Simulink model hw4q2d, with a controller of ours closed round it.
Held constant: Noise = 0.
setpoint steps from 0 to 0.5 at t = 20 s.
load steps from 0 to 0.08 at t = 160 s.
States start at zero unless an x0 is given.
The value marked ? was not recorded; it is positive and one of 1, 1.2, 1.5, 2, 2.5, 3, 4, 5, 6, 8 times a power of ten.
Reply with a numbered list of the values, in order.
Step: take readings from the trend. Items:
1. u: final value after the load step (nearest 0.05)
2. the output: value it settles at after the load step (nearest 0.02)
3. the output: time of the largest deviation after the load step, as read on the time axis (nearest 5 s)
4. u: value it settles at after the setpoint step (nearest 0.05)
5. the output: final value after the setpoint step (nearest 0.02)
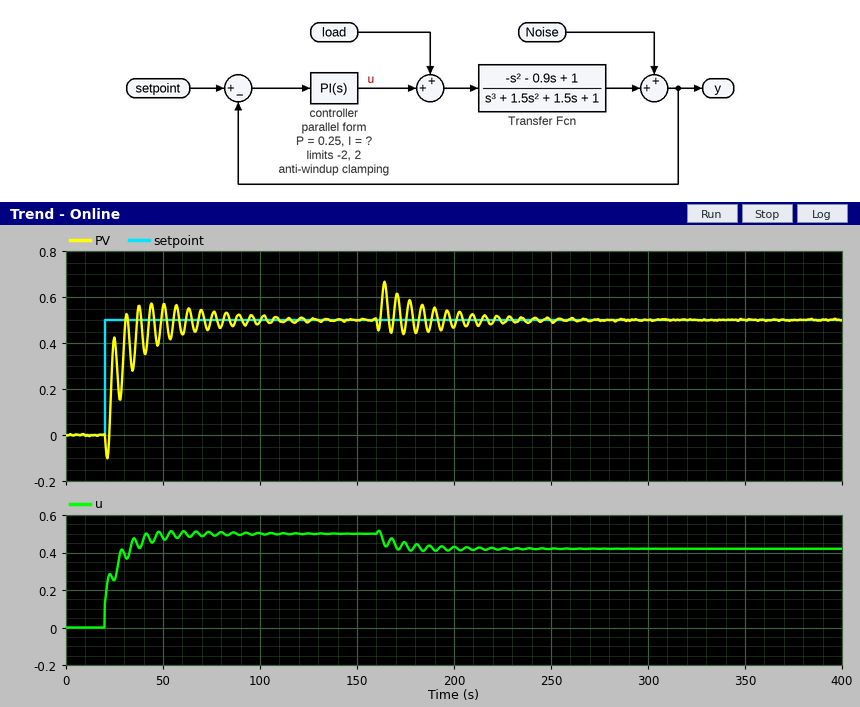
1. 0.40
2. 0.50
3. 165 s
4. 0.50
5. 0.50
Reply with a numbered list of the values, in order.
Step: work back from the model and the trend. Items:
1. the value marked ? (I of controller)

1. 0.12
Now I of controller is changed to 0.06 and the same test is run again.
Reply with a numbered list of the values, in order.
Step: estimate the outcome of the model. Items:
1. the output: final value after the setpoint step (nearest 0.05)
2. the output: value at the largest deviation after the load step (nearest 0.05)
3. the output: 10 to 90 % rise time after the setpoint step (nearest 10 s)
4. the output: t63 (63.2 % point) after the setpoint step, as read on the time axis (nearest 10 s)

1. 0.50
2. 0.65
3. 30 s
4. 30 s
